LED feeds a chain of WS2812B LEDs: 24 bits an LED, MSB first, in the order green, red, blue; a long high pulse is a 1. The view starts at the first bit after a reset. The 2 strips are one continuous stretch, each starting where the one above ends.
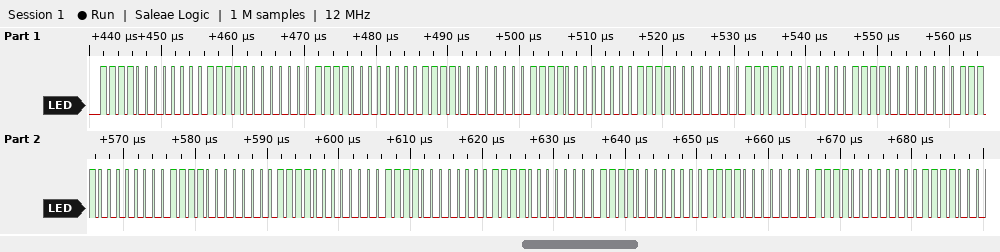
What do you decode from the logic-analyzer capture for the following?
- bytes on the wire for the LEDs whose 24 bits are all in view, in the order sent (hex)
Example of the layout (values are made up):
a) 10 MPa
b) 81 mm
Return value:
a) F0 0F 00 F0 0F 00 F0 0F 00 F0 0F 00 F0 0F 00 F0 0F 00 F0 0F 00 F0 0F 00
